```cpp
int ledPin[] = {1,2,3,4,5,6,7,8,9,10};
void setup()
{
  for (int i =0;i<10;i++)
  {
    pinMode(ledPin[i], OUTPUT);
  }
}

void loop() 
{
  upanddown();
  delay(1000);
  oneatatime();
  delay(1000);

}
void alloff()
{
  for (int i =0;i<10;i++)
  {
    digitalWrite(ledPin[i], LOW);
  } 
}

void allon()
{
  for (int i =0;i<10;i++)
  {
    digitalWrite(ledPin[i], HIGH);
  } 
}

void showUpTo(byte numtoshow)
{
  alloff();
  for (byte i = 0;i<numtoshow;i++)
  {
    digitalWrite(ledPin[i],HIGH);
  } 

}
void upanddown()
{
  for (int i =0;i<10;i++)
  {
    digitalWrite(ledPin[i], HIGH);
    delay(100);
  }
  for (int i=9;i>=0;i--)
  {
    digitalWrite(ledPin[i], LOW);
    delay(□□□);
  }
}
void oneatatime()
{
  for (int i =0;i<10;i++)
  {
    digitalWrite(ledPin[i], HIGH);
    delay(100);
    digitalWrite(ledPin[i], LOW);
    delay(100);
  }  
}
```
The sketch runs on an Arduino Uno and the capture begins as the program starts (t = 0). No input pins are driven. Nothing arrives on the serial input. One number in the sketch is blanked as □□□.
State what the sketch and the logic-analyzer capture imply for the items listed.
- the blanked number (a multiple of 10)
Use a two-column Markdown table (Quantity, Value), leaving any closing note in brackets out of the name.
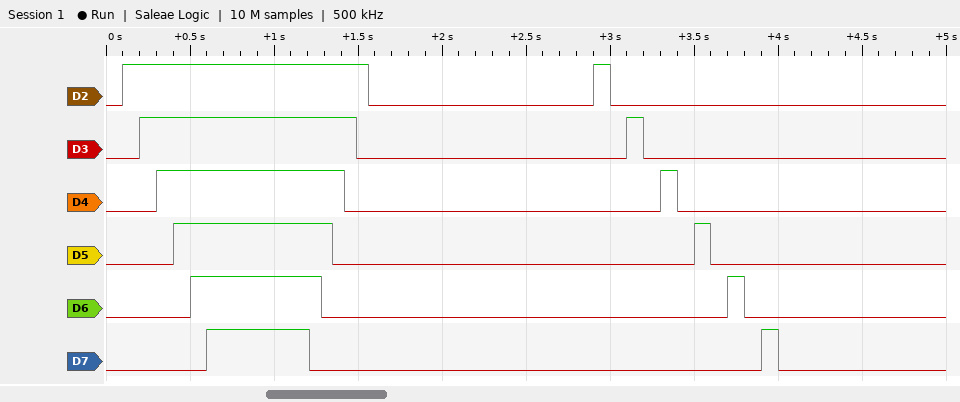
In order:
| Quantity | Value |
|---|---|
| the blanked number | 70 |
